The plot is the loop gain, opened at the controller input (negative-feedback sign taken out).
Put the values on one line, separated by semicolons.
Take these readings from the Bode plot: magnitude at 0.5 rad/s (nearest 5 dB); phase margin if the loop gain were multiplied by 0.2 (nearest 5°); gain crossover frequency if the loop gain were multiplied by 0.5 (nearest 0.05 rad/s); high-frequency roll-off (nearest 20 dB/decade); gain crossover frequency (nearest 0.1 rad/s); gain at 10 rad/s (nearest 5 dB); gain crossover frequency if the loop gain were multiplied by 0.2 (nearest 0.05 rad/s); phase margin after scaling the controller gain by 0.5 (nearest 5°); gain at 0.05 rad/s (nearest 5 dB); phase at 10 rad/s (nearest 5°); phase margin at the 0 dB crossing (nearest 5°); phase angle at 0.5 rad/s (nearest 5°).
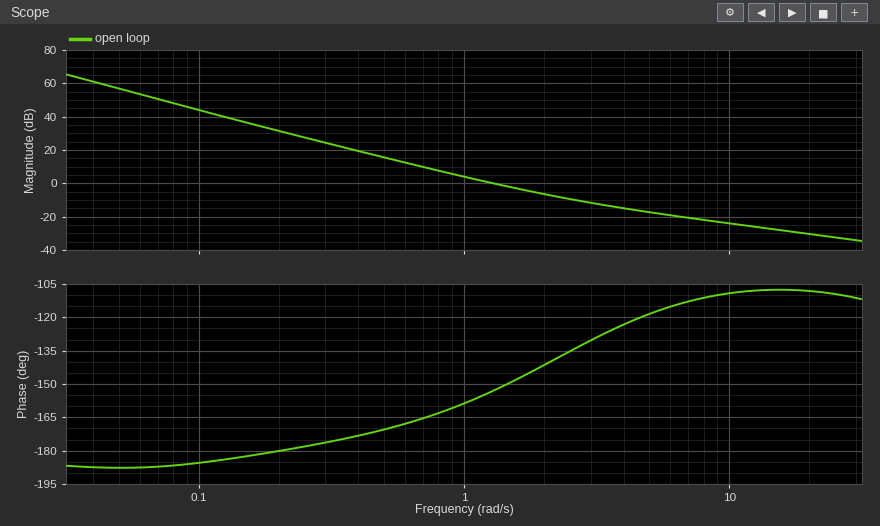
15 dB; 10°; 0.90 rad/s; -20 dB/decade; 1.3 rad/s; -25 dB; 0.55 rad/s; 20°; 55 dB; -110°; 25°; -170°
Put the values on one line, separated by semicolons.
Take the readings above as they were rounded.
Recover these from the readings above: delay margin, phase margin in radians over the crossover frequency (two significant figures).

0.34 s
